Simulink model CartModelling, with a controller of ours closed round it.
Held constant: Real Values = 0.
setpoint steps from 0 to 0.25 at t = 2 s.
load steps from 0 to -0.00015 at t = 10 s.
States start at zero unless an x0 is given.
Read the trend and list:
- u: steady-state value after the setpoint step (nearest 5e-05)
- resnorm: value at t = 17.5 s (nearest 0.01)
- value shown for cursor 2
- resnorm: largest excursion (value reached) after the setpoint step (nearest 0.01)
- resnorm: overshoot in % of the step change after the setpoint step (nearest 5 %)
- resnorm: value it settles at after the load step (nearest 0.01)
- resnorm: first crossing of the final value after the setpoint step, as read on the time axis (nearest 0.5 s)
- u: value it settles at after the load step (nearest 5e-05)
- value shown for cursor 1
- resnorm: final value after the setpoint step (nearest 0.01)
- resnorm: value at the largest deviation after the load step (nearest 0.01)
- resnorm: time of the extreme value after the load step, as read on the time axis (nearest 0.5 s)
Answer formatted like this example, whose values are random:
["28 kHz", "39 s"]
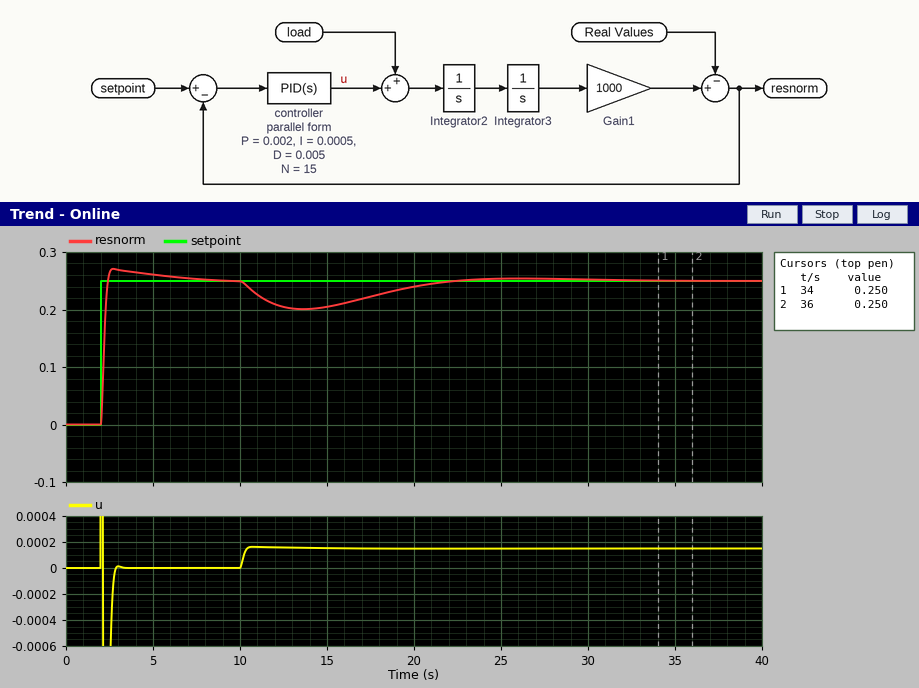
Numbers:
["0.00000", "0.22", "0.250", "0.27", "10 %", "0.25", "2.5 s", "0.00015", "0.250", "0.25", "0.20", "13.5 s"]
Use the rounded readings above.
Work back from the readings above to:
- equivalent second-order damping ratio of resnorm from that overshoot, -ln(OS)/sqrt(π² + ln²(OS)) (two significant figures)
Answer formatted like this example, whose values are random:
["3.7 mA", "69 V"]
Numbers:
["0.59"]
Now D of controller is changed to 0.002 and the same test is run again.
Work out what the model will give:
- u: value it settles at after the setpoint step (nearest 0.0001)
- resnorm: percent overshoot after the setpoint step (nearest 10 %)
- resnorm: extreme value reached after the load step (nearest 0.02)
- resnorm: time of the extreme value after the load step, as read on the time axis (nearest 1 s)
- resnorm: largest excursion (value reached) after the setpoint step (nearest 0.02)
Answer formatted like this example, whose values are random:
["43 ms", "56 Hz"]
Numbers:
["0.0000", "30 %", "0.18", "12 s", "0.32"]
